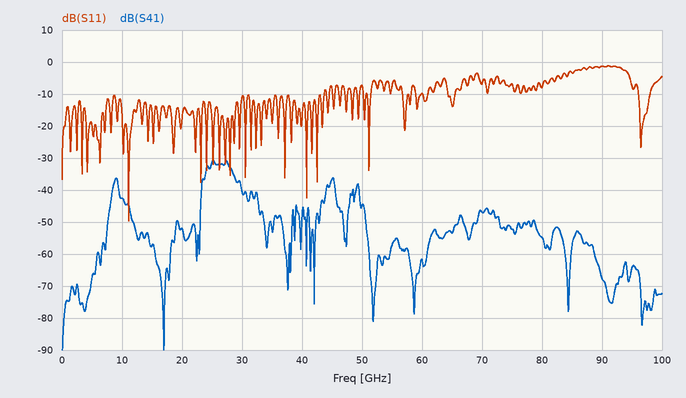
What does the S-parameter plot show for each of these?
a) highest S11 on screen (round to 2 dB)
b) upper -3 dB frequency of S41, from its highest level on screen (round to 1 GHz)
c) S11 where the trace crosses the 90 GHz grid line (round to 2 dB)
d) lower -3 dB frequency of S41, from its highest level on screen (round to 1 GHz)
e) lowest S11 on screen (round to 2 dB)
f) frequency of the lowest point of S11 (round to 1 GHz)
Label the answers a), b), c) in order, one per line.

a) -2 dB
b) 28 GHz
c) -2 dB
d) 24 GHz
e) -50 dB
f) 11 GHz
